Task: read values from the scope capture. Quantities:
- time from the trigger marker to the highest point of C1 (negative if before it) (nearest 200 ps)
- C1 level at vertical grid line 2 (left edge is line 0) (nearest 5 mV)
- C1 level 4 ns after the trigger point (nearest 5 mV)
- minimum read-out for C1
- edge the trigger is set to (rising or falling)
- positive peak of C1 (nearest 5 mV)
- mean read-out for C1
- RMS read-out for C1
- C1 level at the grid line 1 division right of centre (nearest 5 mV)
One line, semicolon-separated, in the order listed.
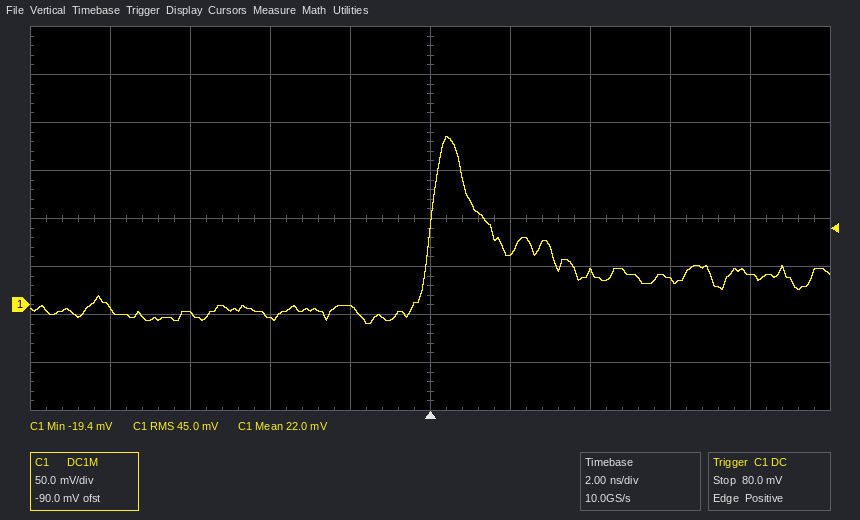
+400 ps; -10 mV; 35 mV; -19.4 mV; rising; 175 mV; 22.0 mV; 45.0 mV; 55 mV
